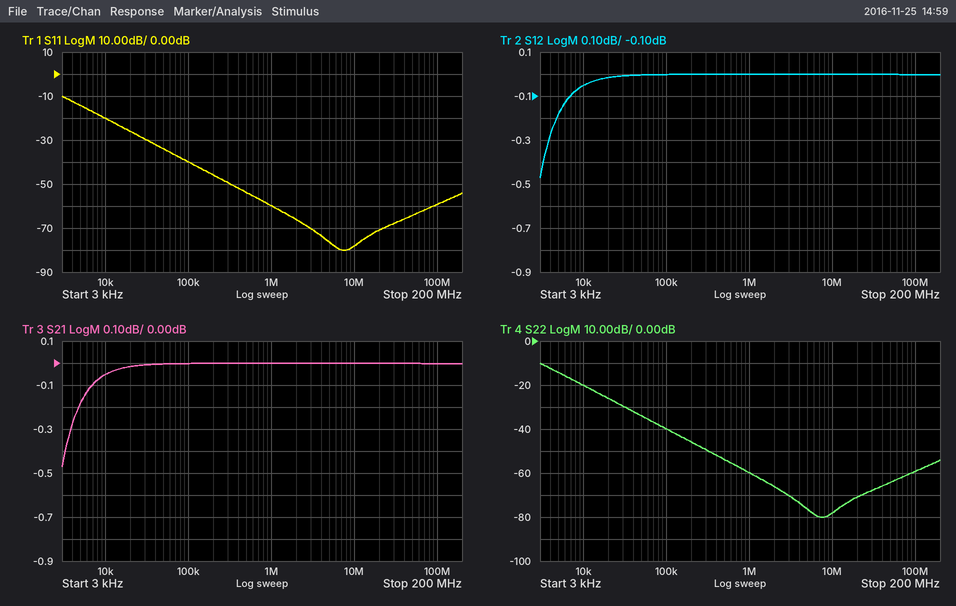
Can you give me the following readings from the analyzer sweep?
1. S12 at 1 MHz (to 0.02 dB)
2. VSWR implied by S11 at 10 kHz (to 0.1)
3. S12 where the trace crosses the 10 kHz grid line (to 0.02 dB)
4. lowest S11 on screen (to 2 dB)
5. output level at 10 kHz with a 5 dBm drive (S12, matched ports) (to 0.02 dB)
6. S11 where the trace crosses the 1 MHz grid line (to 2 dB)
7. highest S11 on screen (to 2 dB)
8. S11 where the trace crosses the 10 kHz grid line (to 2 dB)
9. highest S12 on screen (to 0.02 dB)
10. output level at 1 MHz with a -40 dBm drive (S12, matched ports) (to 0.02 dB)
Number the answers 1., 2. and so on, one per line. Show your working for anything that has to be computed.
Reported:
1. 0.00 dB
2. |Γ| = 10^(-20/20) = 0.1000; VSWR = (1 + 0.1000)/(1 − 0.1000) ≈ 1.2
3. -0.06 dB
4. -80 dB
5. 5 dBm + (-0.06 dB) = 4.94 dBm
6. -60 dB
7. -10 dB
8. -20 dB
9. 0.00 dB
10. -40 dBm + (0.00 dB) = -40.00 dBm
